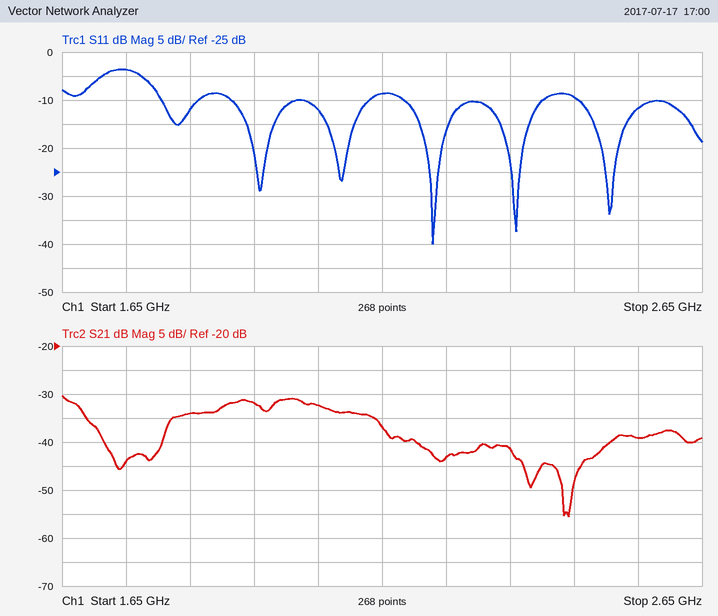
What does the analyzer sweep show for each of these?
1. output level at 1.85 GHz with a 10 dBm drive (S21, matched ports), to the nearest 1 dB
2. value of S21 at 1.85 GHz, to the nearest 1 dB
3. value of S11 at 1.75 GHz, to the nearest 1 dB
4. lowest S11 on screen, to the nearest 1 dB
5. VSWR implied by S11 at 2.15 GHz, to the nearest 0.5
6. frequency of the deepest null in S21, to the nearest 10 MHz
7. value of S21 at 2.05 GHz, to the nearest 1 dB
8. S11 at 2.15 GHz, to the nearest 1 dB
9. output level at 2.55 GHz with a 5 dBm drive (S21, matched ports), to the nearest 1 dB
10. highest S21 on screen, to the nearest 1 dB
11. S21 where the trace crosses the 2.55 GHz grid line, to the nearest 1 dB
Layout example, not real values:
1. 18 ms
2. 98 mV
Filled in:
1. -24 dBm
2. -34 dB
3. -4 dB
4. -40 dB
5. 2.0
6. 2.44 GHz
7. -32 dB
8. -9 dB
9. -34 dBm
10. -30 dB
11. -39 dB
